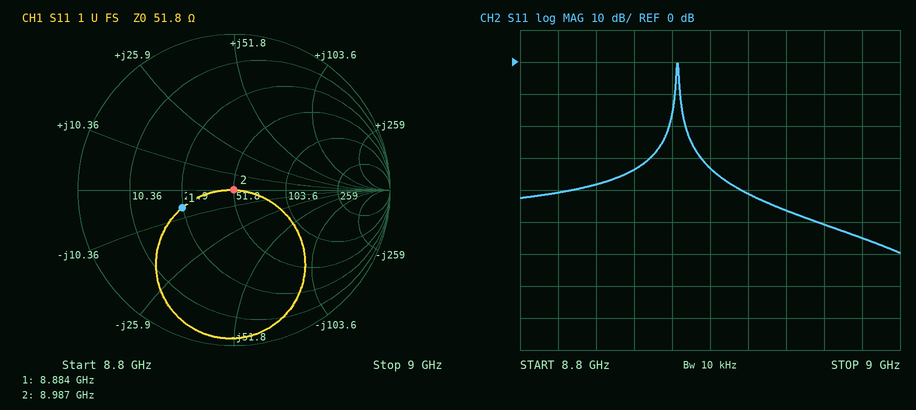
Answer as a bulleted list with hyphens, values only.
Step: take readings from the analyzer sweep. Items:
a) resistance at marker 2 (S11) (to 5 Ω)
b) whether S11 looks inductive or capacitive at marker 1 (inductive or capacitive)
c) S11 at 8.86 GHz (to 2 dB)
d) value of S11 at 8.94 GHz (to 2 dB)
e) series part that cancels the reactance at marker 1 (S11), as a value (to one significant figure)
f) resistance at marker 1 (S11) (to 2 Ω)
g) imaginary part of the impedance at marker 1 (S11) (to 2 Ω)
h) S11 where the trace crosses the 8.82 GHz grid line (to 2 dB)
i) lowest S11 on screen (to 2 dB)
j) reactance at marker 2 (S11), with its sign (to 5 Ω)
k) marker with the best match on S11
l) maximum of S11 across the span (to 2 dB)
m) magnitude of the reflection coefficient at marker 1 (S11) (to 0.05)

- 50 Ω
- capacitive
- -34 dB
- -46 dB
- 100 pH
- 26 Ω
- -6 Ω
- -40 dB
- -60 dB
- 0 Ω
- marker 2
- 0 dB
- 0.35
